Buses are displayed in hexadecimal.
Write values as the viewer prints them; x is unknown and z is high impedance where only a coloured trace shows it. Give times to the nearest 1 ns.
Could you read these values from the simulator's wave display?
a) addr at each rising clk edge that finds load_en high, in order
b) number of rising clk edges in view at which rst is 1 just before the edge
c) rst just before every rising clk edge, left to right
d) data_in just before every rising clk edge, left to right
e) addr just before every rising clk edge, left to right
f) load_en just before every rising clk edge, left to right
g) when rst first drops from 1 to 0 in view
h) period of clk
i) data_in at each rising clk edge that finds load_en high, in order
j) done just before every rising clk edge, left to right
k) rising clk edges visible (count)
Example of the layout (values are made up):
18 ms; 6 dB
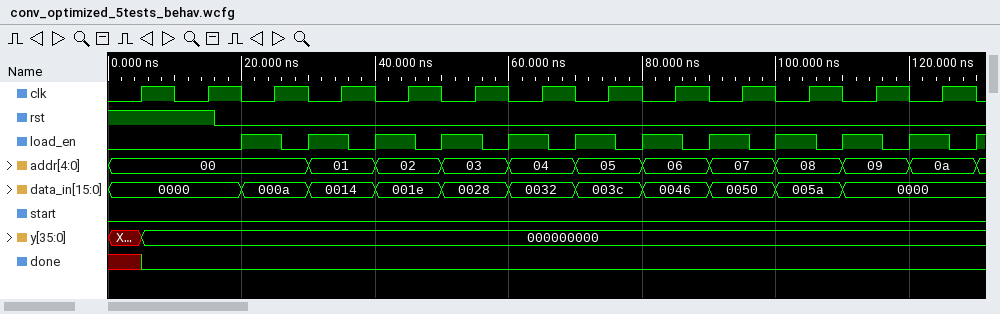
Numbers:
00, 01, 02, 03, 04, 05, 06, 07, 08, 09, 0a; 2; 1 1 0 0 0 0 0 0 0 0 0 0 0; 0000, 0000, 000a, 0014, 001e, 0028, 0032, 003c, 0046, 0050, 005a, 0000, 0000; 00, 00, 00, 01, 02, 03, 04, 05, 06, 07, 08, 09, 0a; 0 0 1 1 1 1 1 1 1 1 1 1 1; 16 ns; 10 ns; 000a, 0014, 001e, 0028, 0032, 003c, 0046, 0050, 005a, 0000, 0000; x 0 0 0 0 0 0 0 0 0 0 0 0; 13
